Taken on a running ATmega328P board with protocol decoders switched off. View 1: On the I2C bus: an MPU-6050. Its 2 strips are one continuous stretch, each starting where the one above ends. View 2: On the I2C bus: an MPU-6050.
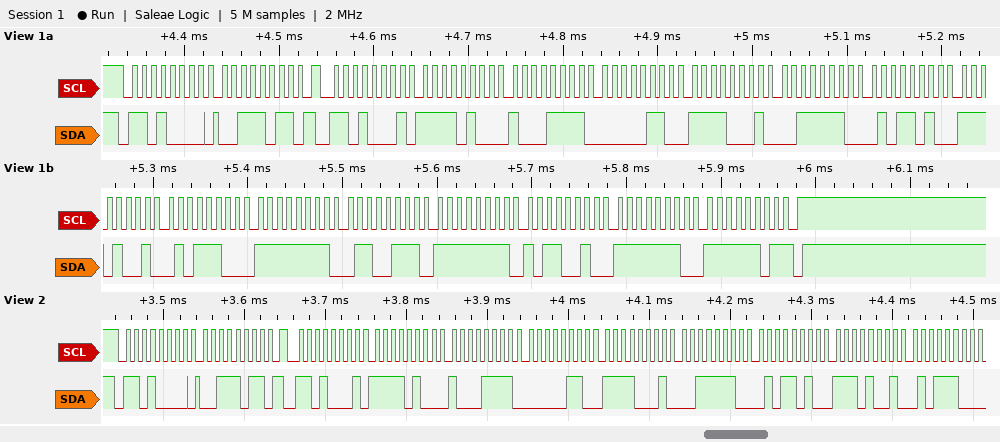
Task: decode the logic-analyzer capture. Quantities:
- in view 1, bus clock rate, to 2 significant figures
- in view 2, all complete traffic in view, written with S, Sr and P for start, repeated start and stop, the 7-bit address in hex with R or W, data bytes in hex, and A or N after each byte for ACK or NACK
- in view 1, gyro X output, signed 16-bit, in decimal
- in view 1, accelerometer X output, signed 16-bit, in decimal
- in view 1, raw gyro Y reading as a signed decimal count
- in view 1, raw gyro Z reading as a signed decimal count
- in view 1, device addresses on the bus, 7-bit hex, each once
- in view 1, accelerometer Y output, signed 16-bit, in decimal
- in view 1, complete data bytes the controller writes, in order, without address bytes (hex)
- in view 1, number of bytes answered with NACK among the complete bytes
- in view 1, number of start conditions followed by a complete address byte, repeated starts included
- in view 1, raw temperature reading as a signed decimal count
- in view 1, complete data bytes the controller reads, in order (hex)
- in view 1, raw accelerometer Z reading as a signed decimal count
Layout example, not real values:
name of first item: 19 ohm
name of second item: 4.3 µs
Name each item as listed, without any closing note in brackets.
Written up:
in view 1, bus clock rate, to 2 significant figures: 100 kHz
in view 2, all complete traffic in view, written with S, Sr and P for start, repeated start and stop, the 7-bit address in hex with R or W, data bytes in hex, and A or N after each byte for ACK or NACK: S 68W A 3B A Sr 68R A F4 A 8F A 06 A F1 A 3E A 5A A E9 A 5C A
in view 1, gyro X output, signed 16-bit, in decimal: -153
in view 1, accelerometer X output, signed 16-bit, in decimal: -2929
in view 1, raw gyro Y reading as a signed decimal count: -78
in view 1, raw gyro Z reading as a signed decimal count: -259
in view 1, device addresses on the bus, 7-bit hex, each once: 0x68
in view 1, accelerometer Y output, signed 16-bit, in decimal: 1777
in view 1, complete data bytes the controller writes, in order, without address bytes: 3B
in view 1, number of bytes answered with NACK among the complete bytes: 1
in view 1, number of start conditions followed by a complete address byte, repeated starts included: 2
in view 1, raw temperature reading as a signed decimal count: -5796
in view 1, complete data bytes the controller reads, in order: F4 8F 06 F1 3E 5A E9 5C FF 67 FF B2 FE FD
in view 1, raw accelerometer Z reading as a signed decimal count: 15962
